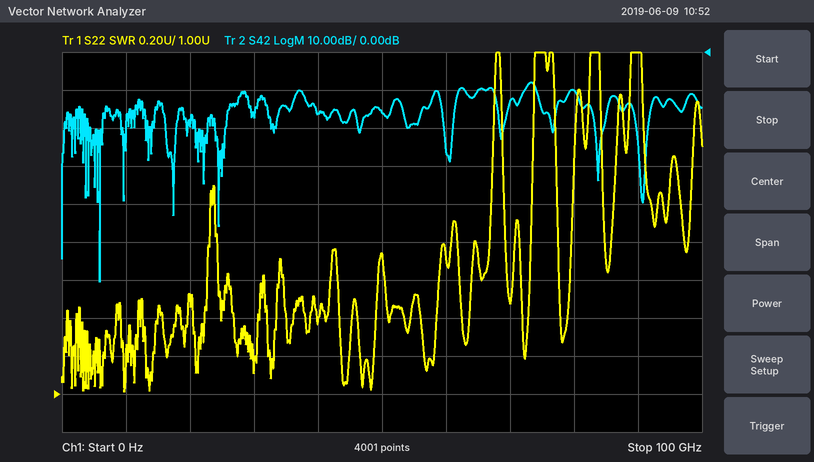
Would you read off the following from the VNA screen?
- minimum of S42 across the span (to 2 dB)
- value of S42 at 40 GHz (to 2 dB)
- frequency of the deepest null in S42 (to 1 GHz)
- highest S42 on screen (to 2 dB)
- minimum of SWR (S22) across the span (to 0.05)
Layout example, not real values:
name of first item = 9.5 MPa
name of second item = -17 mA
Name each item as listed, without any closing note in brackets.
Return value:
minimum of S42 across the span = -60 dB
value of S42 at 40 GHz = -16 dB
frequency of the deepest null in S42 = 6 GHz
highest S42 on screen = -8 dB
minimum of SWR (S22) across the span = 1.00
